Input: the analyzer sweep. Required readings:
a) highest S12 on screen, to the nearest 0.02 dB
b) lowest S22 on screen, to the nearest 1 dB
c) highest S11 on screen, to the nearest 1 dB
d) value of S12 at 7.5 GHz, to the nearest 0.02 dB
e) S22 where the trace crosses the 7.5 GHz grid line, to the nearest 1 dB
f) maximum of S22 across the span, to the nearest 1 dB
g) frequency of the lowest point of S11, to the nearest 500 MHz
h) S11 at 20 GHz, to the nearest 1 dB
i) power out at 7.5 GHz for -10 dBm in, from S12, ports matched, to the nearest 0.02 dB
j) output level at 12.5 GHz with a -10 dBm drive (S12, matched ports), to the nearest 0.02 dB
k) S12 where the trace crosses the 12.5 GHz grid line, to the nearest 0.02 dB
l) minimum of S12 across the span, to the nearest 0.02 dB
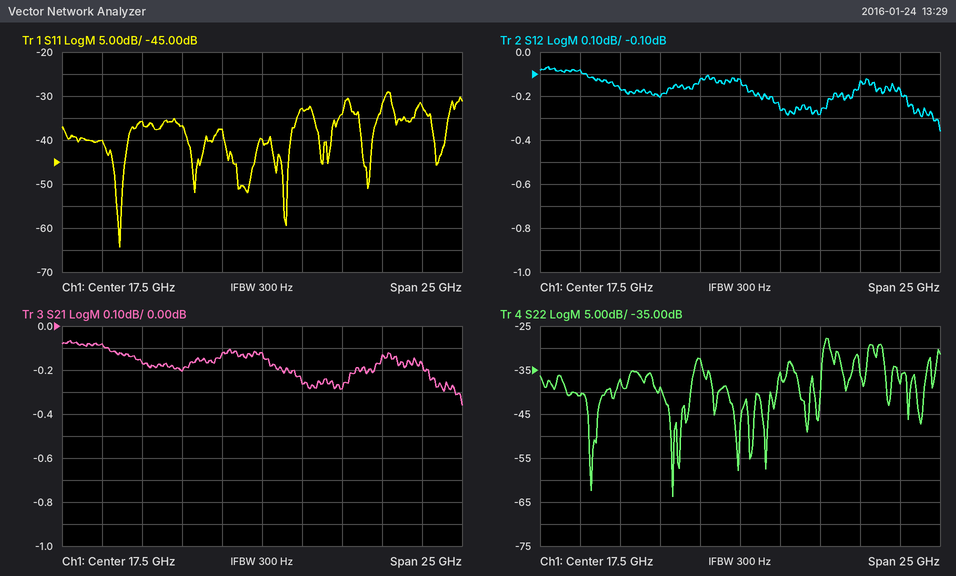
-0.06 dB
-64 dB
-29 dB
-0.08 dB
-41 dB
-28 dB
8.5 GHz
-33 dB
-10.08 dBm
-10.20 dBm
-0.20 dB
-0.36 dB
